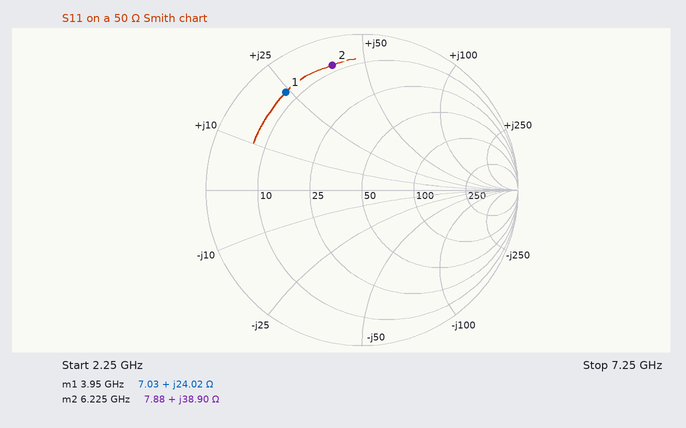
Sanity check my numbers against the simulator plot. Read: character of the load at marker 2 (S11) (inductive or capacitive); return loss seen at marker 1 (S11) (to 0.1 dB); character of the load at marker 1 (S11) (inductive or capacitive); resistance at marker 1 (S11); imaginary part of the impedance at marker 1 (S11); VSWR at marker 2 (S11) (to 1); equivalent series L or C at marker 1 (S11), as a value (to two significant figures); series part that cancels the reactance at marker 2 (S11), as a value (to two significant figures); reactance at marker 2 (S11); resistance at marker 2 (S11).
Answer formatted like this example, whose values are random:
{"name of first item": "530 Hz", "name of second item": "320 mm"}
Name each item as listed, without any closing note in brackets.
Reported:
{"character of the load at marker 2 (S11)": "inductive", "return loss seen at marker 1 (S11)": "2.0 dB", "character of the load at marker 1 (S11)": "inductive", "resistance at marker 1": "7.03 Ω", "imaginary part of the impedance at marker 1": "+24.02 Ω", "VSWR at marker 2 (S11)": "10", "equivalent series L or C at marker 1 (S11), as a value": "970 pH", "series part that cancels the reactance at marker 2 (S11), as a value": "660 fF", "reactance at marker 2": "+38.90 Ω", "resistance at marker 2": "7.88 Ω"}
